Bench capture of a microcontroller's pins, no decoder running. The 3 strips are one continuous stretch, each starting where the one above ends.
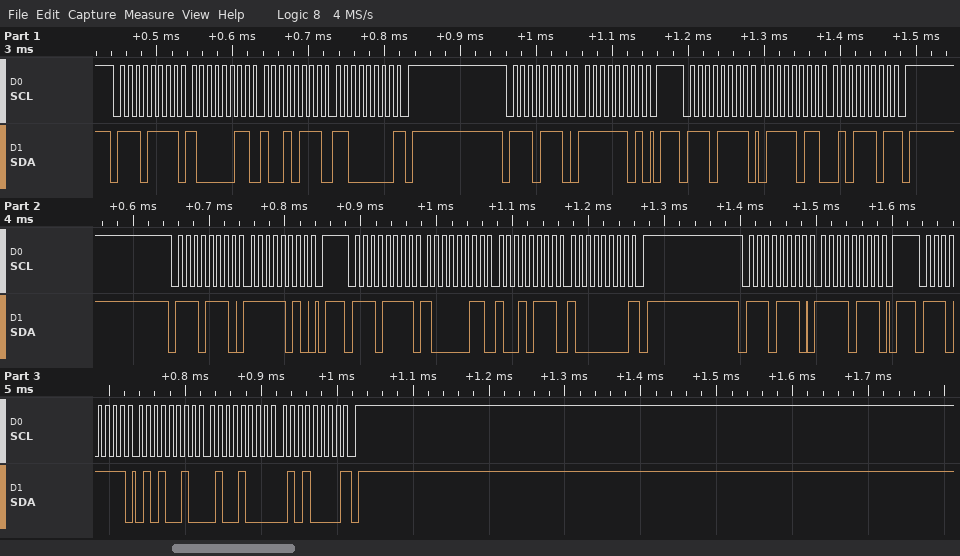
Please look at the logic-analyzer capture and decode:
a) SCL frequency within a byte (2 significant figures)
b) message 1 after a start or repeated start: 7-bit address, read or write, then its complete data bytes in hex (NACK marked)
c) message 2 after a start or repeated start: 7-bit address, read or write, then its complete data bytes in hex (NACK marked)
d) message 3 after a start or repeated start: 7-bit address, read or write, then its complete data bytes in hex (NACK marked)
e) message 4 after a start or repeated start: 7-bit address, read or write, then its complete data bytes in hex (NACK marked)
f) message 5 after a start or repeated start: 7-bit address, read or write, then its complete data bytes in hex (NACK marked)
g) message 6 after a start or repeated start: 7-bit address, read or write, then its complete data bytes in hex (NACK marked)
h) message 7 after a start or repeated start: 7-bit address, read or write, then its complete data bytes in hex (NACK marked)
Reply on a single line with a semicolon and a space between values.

100 kHz; 0x77 read: 83 97 C0 NACK; 0x77 write: FD; 0x77 read: 7B 5D NACK; 0x77 write: FA; 0x77 read: 83 97 80 NACK; 0x77 write: F7; 0x77 read: 52 48 50 NACK
